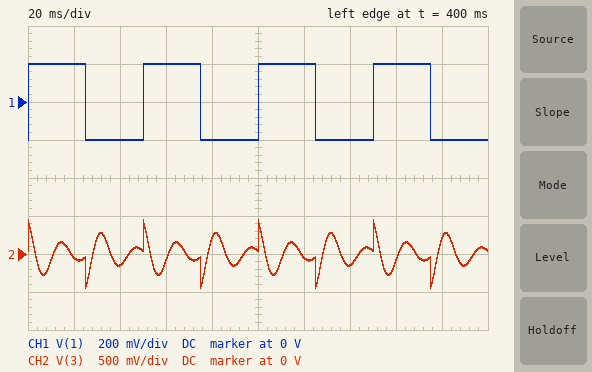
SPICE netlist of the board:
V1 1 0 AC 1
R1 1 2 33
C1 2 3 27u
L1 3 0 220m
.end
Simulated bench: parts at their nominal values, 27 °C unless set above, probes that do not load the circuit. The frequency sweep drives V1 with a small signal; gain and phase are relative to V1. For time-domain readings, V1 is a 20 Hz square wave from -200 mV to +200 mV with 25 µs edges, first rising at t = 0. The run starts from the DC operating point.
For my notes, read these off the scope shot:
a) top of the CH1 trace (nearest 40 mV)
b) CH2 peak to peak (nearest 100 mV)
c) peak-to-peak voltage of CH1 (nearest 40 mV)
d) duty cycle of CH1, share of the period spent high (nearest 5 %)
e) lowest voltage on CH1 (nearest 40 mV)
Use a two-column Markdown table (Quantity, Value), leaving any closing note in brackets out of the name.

| Quantity | Value |
|---|---|
| top of the CH1 trace | 200 mV |
| CH2 peak to peak | 900 mV |
| peak-to-peak voltage of CH1 | 400 mV |
| duty cycle of CH1, share of the period spent high | 50 % |
| lowest voltage on CH1 | -200 mV |
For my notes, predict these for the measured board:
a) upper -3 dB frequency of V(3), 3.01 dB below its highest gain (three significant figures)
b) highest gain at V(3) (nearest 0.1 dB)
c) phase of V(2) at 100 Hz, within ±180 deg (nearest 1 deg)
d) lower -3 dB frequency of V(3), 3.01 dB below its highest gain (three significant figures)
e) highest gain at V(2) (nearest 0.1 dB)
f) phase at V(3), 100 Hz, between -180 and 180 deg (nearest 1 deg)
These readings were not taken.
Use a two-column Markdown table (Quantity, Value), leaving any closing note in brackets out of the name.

| Quantity | Value |
|---|---|
| upper -3 dB frequency of V(3), 3.01 dB below its highest gain | 86.2 Hz |
| highest gain at V(3) | 8.9 dB |
| phase of V(2) at 100 Hz, within ±180 deg | 23 deg |
| lower -3 dB frequency of V(3), 3.01 dB below its highest gain | 57.4 Hz |
| highest gain at V(2) | 0 dB |
| phase at V(3), 100 Hz, between -180 and 180 deg | 23 deg |
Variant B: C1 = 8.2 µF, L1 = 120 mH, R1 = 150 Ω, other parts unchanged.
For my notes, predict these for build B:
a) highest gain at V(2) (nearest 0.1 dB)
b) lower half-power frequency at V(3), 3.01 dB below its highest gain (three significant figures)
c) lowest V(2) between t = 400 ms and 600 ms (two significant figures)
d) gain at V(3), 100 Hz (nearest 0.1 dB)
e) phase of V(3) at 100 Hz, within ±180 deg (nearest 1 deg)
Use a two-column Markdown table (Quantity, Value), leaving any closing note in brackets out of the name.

| Quantity | Value |
|---|---|
| highest gain at V(2) | 0 dB |
| lower half-power frequency at V(3), 3.01 dB below its highest gain | 146 Hz |
| lowest V(2) between t = 400 ms and 600 ms | -220 mV |
| gain at V(3), 100 Hz | -8.1 dB |
| phase of V(3) at 100 Hz, within ±180 deg | 128 deg |
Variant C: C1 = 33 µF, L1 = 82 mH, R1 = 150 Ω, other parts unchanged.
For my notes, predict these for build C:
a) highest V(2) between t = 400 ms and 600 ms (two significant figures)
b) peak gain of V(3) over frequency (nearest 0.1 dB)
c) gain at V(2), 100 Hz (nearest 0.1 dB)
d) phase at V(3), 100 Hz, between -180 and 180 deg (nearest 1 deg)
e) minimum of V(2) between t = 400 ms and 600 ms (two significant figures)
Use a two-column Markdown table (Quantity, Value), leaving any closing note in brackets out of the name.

| Quantity | Value |
|---|---|
| highest V(2) between t = 400 ms and 600 ms | 200 mV |
| peak gain of V(3) over frequency | 0 dB |
| gain at V(2), 100 Hz | -33.2 dB |
| phase at V(3), 100 Hz, between -180 and 180 deg | 89 deg |
| minimum of V(2) between t = 400 ms and 600 ms | -200 mV |
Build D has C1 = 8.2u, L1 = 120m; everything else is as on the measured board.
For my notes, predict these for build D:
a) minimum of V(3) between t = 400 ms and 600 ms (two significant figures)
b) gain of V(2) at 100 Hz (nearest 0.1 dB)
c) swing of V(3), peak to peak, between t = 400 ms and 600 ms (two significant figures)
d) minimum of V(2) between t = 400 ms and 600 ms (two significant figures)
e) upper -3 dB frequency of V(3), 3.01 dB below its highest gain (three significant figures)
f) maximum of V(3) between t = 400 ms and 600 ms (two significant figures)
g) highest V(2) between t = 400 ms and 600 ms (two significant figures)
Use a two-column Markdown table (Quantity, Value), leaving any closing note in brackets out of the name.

| Quantity | Value |
|---|---|
| minimum of V(3) between t = 400 ms and 600 ms | -390 mV |
| gain of V(2) at 100 Hz | -0.3 dB |
| swing of V(3), peak to peak, between t = 400 ms and 600 ms | 770 mV |
| minimum of V(2) between t = 400 ms and 600 ms | -260 mV |
| upper -3 dB frequency of V(3), 3.01 dB below its highest gain | 193 Hz |
| maximum of V(3) between t = 400 ms and 600 ms | 390 mV |
| highest V(2) between t = 400 ms and 600 ms | 260 mV |
